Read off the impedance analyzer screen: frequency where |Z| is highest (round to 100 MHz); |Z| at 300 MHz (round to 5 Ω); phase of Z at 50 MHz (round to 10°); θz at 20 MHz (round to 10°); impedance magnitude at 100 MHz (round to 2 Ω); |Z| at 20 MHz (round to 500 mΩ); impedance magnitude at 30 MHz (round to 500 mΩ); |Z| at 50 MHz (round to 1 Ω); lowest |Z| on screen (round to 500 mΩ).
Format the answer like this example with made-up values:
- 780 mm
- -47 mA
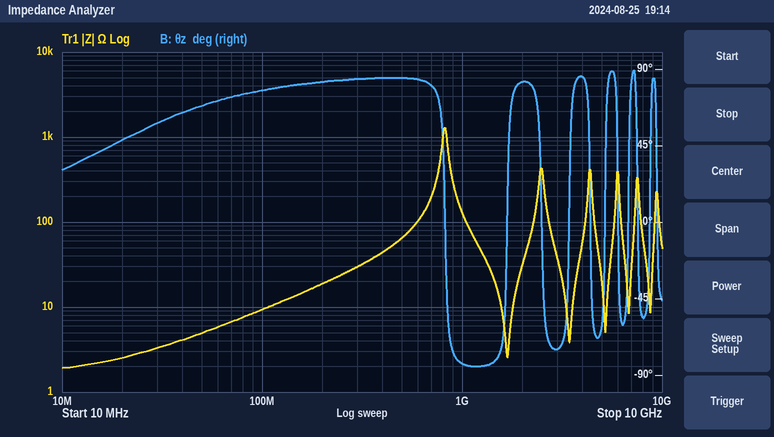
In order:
- 800 MHz
- 30 Ω
- 70°
- 50°
- 10 Ω
- 2.5 Ω
- 3.5 Ω
- 5 Ω
- 2.0 Ω
